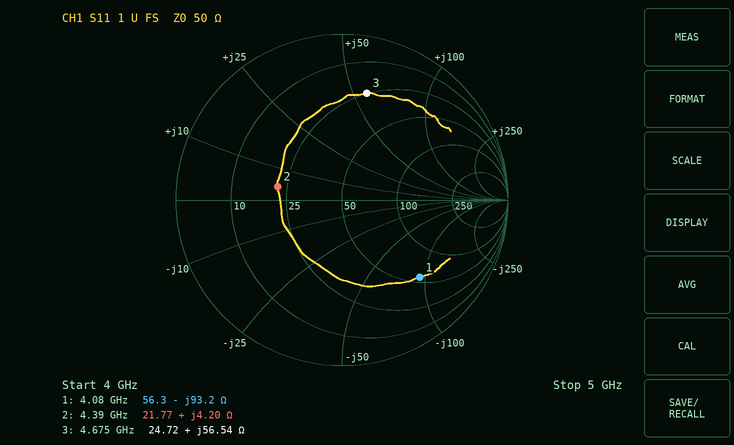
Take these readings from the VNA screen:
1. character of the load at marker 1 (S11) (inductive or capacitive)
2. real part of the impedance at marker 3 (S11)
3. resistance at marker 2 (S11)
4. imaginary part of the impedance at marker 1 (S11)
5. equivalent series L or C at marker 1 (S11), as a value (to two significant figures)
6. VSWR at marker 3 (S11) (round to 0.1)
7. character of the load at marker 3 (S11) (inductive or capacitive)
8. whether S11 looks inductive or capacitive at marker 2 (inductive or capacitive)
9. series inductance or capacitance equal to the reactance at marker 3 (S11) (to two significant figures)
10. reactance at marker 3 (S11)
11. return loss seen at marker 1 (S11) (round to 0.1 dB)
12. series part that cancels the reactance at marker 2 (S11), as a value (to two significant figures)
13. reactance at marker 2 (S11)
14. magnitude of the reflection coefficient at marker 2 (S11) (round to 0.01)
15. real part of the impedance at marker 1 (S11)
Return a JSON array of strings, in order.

["capacitive", "24.72 Ω", "21.77 Ω", "-93.2 Ω", "420 fF", "4.9", "inductive", "inductive", "1.9 nH", "+56.54 Ω", "3.6 dB", "8.6 pF", "+4.20 Ω", "0.40", "56.3 Ω"]
